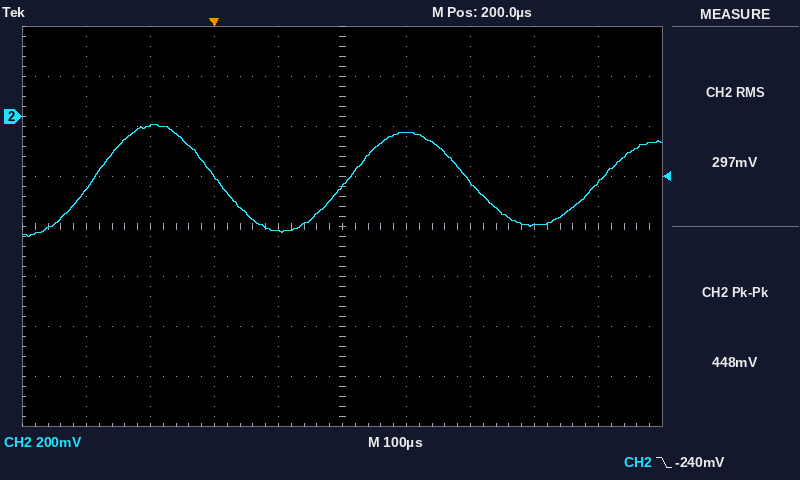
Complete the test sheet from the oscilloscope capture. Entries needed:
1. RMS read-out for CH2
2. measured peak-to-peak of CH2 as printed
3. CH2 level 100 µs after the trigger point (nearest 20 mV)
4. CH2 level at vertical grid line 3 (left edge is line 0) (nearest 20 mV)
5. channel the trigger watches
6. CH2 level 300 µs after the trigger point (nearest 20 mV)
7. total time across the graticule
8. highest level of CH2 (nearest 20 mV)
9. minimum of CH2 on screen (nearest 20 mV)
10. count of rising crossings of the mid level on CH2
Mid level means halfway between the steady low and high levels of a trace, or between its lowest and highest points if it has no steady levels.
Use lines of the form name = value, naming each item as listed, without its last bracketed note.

RMS read-out for CH2 = 297 mV
measured peak-to-peak of CH2 as printed = 448 mV
CH2 level 100 µs after the trigger point = -460 mV
CH2 level at vertical grid line 3 (left edge is line 0) = -240 mV
channel the trigger watches = CH2
CH2 level 300 µs after the trigger point = -60 mV
total time across the graticule = 1 ms
highest level of CH2 = -40 mV
minimum of CH2 on screen = -480 mV
count of rising crossings of the mid level on CH2 = 3
